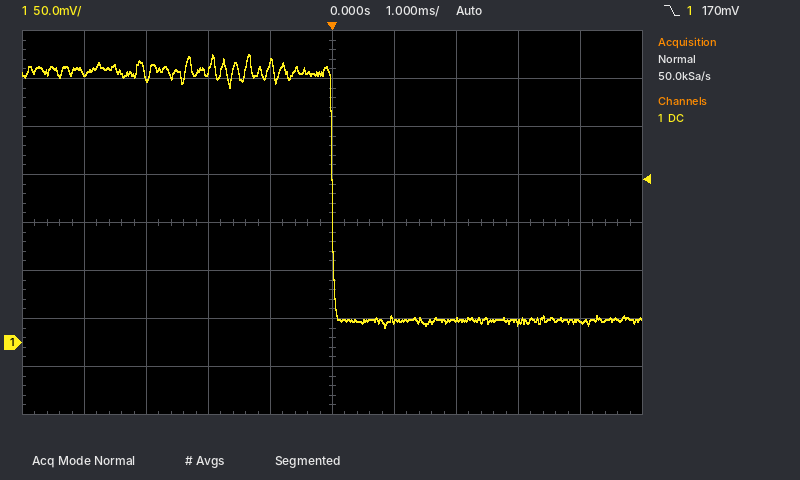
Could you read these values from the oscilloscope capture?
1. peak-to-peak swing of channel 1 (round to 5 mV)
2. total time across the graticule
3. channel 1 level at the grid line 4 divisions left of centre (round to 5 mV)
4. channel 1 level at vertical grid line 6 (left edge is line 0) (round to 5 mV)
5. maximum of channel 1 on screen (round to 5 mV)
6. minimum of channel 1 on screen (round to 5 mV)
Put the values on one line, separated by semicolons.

285 mV; 10 ms; 280 mV; 25 mV; 300 mV; 15 mV
